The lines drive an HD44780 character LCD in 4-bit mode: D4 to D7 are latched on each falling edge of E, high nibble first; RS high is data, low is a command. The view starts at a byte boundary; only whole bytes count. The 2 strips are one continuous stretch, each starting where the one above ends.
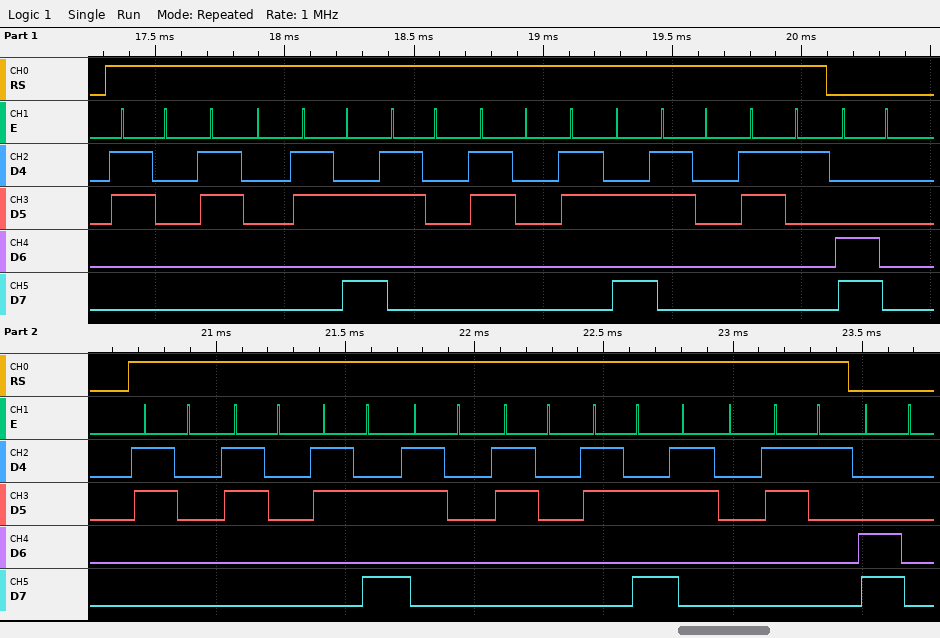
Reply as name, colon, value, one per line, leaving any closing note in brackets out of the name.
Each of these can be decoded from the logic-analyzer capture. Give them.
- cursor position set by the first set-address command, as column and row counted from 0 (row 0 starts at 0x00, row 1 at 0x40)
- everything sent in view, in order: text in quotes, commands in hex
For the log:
cursor position set by the first set-address command, as column and row counted from 0: column 0, row 1
everything sent in view, in order: text in quotes, commands in hex: "00:00:01" 0xC0 "00:00:01" 0xC0
